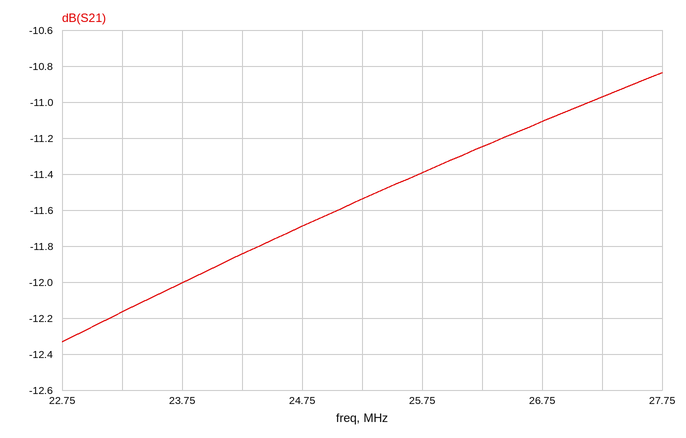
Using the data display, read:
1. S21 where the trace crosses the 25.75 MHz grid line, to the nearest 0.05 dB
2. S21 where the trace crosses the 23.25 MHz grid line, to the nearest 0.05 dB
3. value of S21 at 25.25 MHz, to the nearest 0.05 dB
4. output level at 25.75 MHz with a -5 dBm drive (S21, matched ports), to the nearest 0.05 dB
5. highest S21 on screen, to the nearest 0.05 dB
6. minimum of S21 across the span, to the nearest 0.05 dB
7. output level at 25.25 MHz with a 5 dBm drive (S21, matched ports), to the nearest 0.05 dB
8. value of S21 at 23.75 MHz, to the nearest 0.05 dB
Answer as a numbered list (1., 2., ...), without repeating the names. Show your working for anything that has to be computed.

1. -11.40 dB
2. -12.15 dB
3. -11.55 dB
4. -5 dBm + (-11.40 dB) = -16.40 dBm
5. -10.85 dB
6. -12.35 dB
7. 5 dBm + (-11.55 dB) = -6.55 dBm
8. -12.00 dB
